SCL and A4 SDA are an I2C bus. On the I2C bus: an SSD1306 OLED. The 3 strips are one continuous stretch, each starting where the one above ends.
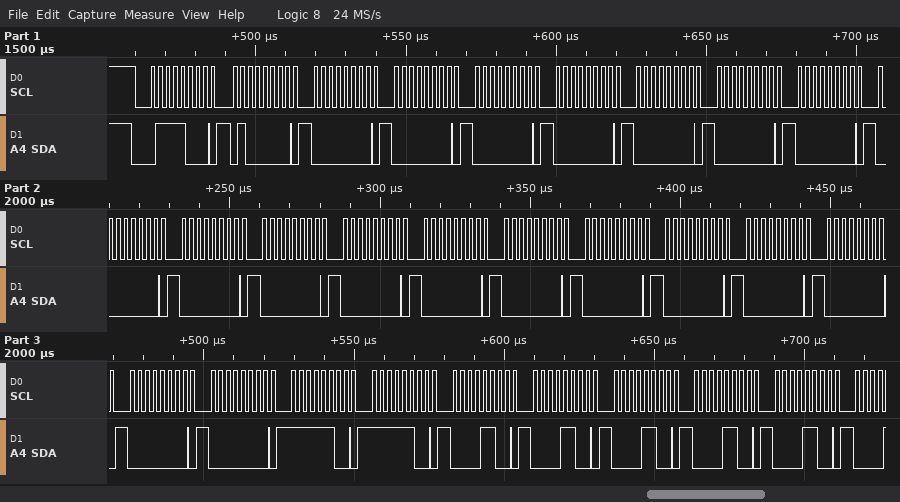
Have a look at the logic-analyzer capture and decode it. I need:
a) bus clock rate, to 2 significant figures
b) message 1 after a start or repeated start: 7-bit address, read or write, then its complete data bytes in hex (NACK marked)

400 kHz
0x3C write: 40 00 00 00 00 00 00 00 00 00 00 00 00 00 00 00 00 00 00 00 FC FC 0C 0C 0C 0C 0C
